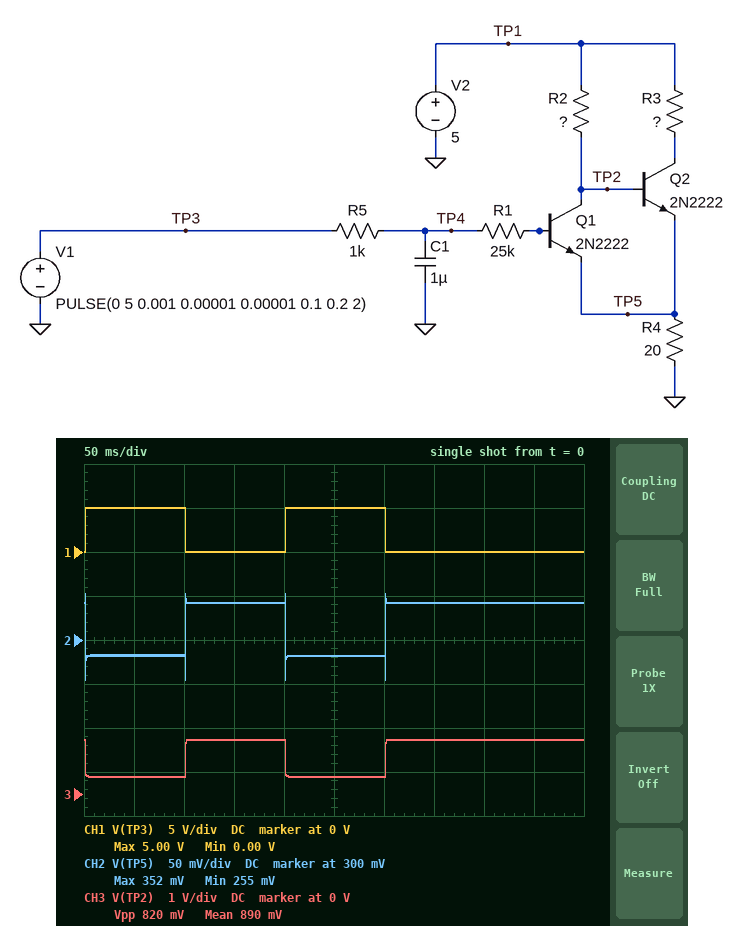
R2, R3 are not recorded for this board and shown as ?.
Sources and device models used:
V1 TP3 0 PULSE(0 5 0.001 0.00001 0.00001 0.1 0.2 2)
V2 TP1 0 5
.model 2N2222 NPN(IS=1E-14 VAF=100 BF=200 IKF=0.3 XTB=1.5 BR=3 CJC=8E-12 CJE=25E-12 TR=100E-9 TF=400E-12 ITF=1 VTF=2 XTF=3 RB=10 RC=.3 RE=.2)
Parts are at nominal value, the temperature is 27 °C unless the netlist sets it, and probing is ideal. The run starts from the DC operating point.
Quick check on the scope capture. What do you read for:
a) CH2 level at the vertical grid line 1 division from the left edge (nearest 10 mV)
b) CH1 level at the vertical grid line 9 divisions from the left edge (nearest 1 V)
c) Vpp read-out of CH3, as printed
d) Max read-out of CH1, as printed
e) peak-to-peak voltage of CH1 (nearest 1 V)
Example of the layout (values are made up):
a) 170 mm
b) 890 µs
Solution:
a) 280 mV
b) 0 V
c) 820 mV
d) 5.00 V
e) 5 V
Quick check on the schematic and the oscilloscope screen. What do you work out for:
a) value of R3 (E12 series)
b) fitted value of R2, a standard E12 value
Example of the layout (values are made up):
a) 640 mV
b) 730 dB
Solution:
a) 820 Ω
b) 330 Ω
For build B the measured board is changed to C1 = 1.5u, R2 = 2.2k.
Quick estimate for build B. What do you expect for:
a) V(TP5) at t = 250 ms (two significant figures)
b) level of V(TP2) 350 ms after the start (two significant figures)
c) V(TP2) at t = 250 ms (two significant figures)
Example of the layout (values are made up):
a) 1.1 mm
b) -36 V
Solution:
a) 48 mV
b) 900 mV
c) 97 mV
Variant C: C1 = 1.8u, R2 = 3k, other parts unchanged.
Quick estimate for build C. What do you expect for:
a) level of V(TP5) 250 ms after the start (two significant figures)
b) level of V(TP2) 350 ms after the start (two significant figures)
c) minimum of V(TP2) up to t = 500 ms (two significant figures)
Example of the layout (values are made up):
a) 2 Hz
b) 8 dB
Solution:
a) 36 mV
b) 880 mV
c) 78 mV
